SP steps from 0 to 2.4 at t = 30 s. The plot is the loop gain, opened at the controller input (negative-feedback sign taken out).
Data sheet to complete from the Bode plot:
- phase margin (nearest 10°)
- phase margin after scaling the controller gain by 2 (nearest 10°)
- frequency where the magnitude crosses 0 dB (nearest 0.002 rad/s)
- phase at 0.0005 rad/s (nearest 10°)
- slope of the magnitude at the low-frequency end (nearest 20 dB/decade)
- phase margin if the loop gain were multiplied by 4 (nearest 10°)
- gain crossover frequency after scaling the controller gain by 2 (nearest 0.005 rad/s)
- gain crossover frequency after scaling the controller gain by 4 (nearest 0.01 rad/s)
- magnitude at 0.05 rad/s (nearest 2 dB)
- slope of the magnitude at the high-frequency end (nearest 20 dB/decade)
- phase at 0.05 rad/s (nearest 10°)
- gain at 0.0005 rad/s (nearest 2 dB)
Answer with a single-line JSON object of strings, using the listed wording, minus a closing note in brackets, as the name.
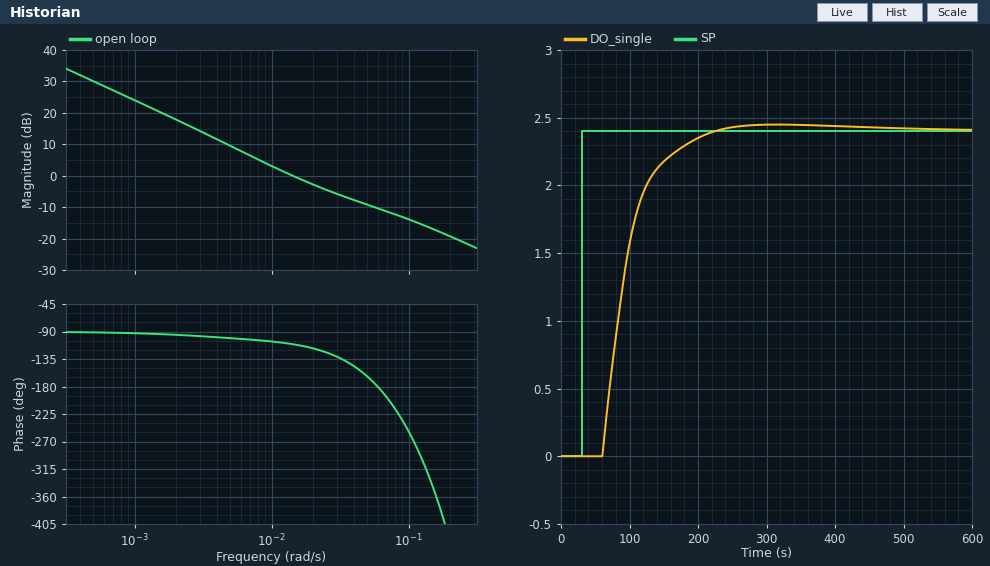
{"phase margin": "70°", "phase margin after scaling the controller gain by 2": "50°", "frequency where the magnitude crosses 0 dB": "0.014 rad/s", "phase at 0.0005 rad/s": "-90°", "slope of the magnitude at the low-frequency end": "-20 dB/decade", "phase margin if the loop gain were multiplied by 4": "-30°", "gain crossover frequency after scaling the controller gain by 2": "0.030 rad/s", "gain crossover frequency after scaling the controller gain by 4": "0.08 rad/s", "magnitude at 0.05 rad/s": "-10 dB", "slope of the magnitude at the high-frequency end": "-20 dB/decade", "phase at 0.05 rad/s": "-160°", "gain at 0.0005 rad/s": "30 dB"}
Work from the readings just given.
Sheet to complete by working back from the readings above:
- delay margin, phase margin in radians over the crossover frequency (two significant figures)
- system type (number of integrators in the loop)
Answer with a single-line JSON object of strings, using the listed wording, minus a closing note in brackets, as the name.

{"delay margin, phase margin in radians over the crossover frequency": "87 s", "system type": "1"}
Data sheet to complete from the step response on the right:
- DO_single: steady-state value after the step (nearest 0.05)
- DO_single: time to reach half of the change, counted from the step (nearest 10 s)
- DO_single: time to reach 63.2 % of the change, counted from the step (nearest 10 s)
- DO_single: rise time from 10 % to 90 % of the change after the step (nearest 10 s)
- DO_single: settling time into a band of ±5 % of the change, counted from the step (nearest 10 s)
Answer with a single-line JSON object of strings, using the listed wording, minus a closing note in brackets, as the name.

{"DO_single: steady-state value after the step": "2.40", "DO_single: time to reach half of the change, counted from the step": "60 s", "DO_single: time to reach 63.2 % of the change, counted from the step": "70 s", "DO_single: rise time from 10 % to 90 % of the change after the step": "80 s", "DO_single: settling time into a band of ±5 % of the change, counted from the step": "150 s"}
